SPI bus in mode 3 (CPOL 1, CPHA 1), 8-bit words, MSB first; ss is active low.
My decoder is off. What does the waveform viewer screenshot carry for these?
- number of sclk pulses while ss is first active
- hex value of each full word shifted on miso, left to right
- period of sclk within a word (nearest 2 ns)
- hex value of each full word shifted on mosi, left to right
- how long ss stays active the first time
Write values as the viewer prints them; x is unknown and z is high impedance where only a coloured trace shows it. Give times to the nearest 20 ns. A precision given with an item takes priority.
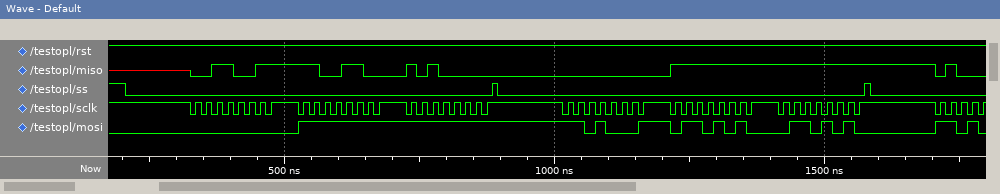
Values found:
24
33, CC, A0, 00, FF, FF
20 ns
00, FF, FF, D1, 6A, 6A
680 ns
